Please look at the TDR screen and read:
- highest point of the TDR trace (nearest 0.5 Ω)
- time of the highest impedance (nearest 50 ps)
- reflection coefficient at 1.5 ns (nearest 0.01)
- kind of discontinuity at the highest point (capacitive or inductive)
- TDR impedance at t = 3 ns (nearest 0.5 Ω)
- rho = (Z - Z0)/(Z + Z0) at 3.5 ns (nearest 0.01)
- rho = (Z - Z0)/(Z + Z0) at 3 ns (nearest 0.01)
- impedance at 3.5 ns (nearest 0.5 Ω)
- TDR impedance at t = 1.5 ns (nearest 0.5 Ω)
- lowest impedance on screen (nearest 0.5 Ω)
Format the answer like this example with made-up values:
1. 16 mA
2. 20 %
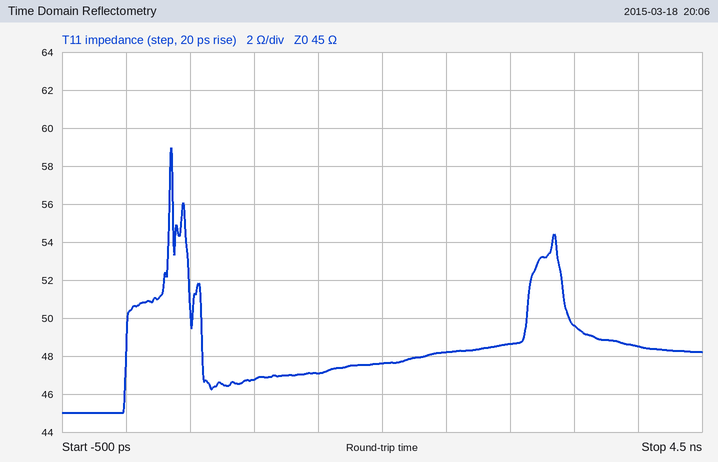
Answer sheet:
1. 59.0 Ω
2. 350 ps
3. +0.02
4. inductive
5. 48.5 Ω
6. +0.05
7. +0.04
8. 49.5 Ω
9. 47.0 Ω
10. 45.0 Ω
